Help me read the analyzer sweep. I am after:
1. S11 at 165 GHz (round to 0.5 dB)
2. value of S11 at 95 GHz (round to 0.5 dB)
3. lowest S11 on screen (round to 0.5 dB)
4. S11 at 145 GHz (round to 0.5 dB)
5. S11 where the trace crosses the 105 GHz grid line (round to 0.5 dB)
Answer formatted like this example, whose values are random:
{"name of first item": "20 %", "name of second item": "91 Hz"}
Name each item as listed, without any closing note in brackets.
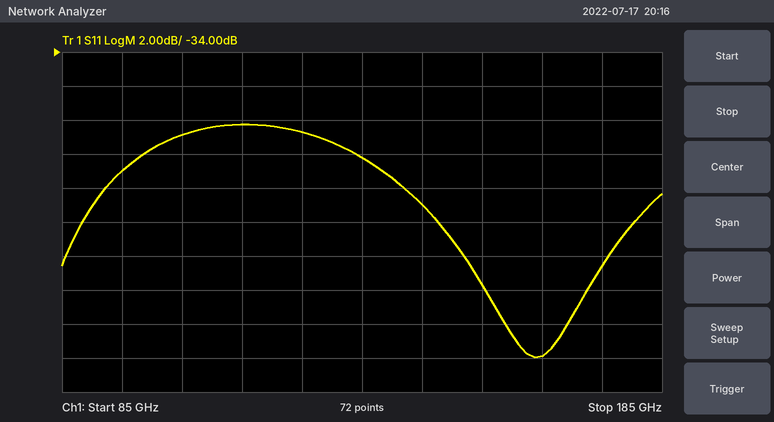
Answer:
{"S11 at 165 GHz": "-52.0 dB", "value of S11 at 95 GHz": "-41.0 dB", "lowest S11 on screen": "-52.0 dB", "S11 at 145 GHz": "-43.0 dB", "S11 where the trace crosses the 105 GHz grid line": "-39.0 dB"}
